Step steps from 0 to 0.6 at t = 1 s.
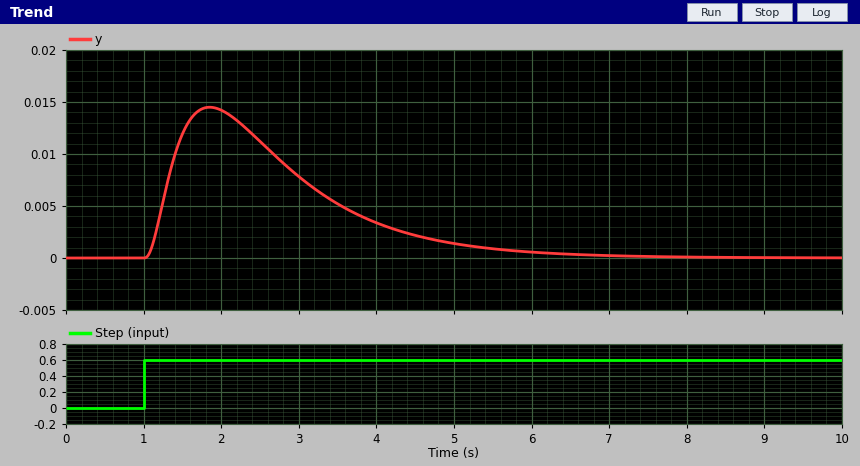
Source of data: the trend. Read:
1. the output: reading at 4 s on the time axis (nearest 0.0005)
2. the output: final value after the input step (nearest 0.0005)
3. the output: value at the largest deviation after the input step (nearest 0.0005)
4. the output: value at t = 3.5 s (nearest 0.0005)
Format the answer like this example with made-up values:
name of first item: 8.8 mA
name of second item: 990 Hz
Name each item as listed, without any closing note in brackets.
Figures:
the output: reading at 4 s on the time axis: 0.0035
the output: final value after the input step: 0.0000
the output: value at the largest deviation after the input step: 0.0145
the output: value at t = 3.5 s: 0.0050
